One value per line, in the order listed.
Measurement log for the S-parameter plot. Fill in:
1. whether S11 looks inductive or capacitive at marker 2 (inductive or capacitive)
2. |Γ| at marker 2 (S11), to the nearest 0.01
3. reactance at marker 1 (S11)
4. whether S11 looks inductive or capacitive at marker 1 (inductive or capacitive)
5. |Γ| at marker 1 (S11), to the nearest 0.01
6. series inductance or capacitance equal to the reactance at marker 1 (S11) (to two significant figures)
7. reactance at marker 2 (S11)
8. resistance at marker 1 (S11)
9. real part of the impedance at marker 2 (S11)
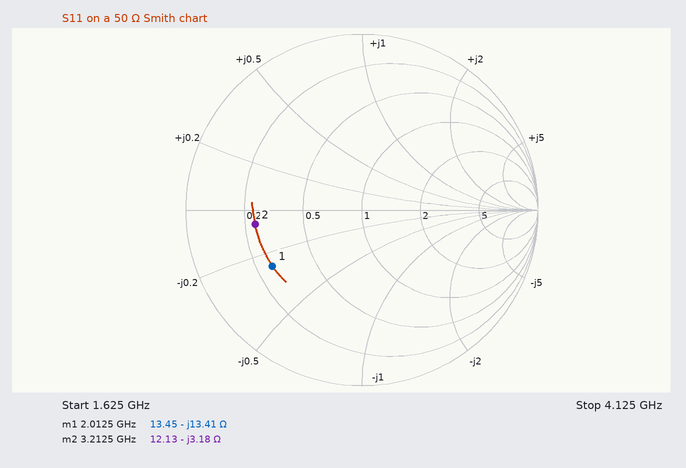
capacitive
0.61
-13.41 Ω
capacitive
0.60
5.9 pF
-3.18 Ω
13.45 Ω
12.13 Ω
